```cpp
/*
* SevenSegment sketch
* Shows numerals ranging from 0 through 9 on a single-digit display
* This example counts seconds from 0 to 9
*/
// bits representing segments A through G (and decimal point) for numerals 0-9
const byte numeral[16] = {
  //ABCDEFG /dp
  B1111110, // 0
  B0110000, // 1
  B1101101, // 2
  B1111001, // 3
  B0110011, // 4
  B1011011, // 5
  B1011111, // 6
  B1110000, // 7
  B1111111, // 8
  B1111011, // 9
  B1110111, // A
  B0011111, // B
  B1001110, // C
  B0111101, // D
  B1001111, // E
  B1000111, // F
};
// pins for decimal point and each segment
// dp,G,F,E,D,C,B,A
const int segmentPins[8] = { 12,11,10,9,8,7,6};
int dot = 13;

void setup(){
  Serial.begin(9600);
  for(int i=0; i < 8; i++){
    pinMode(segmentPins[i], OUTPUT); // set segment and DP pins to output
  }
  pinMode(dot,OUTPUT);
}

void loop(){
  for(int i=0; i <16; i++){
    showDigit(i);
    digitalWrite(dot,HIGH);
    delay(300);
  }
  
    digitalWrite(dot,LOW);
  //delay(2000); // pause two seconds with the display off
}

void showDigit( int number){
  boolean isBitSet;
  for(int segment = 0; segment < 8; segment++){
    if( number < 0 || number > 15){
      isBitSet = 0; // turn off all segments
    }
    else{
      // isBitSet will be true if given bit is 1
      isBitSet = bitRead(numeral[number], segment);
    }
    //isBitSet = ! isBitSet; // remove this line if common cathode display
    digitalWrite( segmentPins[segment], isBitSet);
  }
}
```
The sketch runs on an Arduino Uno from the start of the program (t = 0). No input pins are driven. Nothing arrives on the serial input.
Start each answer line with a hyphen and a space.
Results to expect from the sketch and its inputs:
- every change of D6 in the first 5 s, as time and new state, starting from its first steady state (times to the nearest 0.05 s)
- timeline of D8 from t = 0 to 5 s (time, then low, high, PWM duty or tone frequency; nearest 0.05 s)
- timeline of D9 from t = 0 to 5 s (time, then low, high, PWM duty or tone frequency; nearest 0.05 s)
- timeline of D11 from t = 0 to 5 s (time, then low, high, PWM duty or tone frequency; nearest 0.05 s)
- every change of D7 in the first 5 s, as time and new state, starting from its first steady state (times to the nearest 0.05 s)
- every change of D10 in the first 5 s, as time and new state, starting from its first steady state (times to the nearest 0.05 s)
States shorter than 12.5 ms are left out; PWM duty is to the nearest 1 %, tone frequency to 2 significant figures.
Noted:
- 0 s high; 0.3 s low; 0.6 s high; 1.2 s low; 1.5 s high; 3.3 s low; 3.6 s high; 3.9 s low; 4.2 s high
- 0 s high; 0.6 s low; 0.9 s high; 3.6 s low; 3.9 s high; 4.2 s low; 4.8 s high
- 0 s high; 0.3 s low; 0.6 s high; 1.2 s low; 1.5 s high; 2.1 s low; 2.4 s high; 3 s low; 3.3 s high; 4.5 s low; 4.8 s high
- 0 s high; 0.3 s low; 1.2 s high; 2.1 s low; 2.4 s high; 3.9 s low; 4.2 s high
- 0 s high; 1.5 s low; 2.1 s high; 3.3 s low; 3.9 s high; 4.2 s low; 4.8 s high
- 0 s high; 0.3 s low; 0.6 s high; 0.9 s low; 1.8 s high; 2.1 s low; 2.4 s high; 2.7 s low; 3 s high
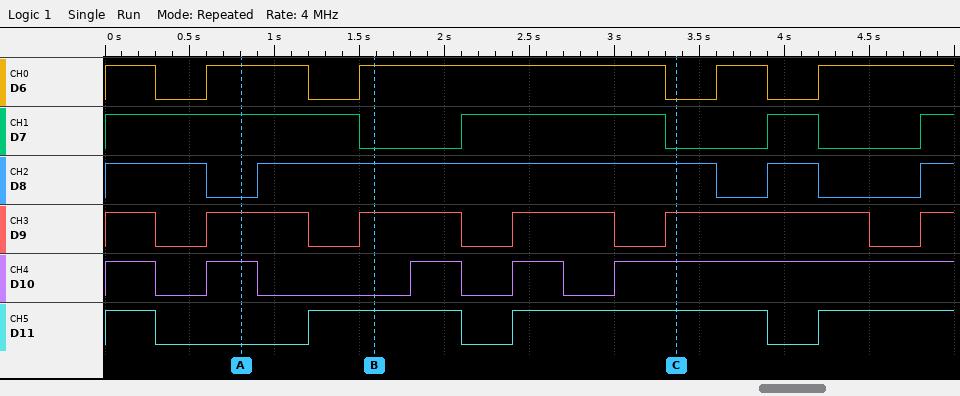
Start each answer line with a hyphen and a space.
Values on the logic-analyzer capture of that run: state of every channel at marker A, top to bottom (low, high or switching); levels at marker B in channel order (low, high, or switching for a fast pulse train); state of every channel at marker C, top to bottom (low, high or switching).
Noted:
- D6 high, D7 high, D8 low, D9 high, D10 high, D11 low
- D6 high, D7 low, D8 high, D9 high, D10 low, D11 high
- D6 low, D7 low, D8 high, D9 high, D10 high, D11 high
